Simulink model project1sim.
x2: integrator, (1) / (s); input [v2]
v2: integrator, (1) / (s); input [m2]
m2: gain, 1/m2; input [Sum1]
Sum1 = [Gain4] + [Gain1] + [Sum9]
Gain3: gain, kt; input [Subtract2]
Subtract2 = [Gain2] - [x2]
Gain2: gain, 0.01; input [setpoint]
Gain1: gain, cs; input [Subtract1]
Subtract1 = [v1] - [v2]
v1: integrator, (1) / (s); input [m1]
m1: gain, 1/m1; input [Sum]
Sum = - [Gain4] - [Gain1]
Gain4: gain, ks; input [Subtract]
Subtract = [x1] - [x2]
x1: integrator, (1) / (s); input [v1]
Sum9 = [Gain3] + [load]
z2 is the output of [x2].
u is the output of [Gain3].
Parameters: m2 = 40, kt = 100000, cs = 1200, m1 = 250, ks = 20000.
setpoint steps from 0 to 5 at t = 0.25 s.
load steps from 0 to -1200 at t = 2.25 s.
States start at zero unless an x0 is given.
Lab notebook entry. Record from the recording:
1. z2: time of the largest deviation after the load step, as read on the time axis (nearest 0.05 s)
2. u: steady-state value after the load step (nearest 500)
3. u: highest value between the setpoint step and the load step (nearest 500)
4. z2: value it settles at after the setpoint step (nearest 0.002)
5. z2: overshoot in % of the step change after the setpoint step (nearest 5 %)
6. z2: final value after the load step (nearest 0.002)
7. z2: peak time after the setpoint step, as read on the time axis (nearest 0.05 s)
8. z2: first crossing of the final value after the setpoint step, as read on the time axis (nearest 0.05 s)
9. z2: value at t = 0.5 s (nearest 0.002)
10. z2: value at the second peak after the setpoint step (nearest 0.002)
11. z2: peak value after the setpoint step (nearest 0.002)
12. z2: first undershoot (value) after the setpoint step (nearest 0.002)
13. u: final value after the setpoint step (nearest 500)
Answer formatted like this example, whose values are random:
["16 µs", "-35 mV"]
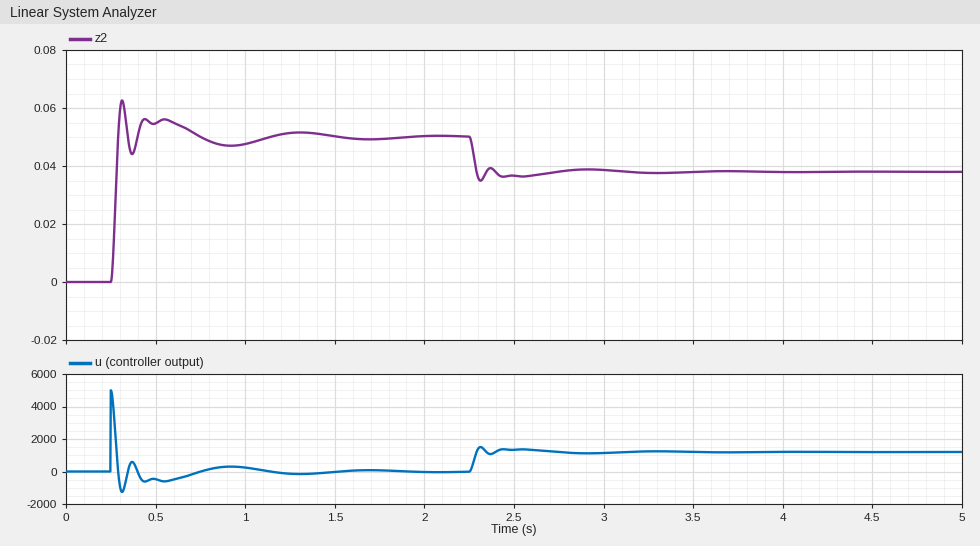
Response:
["2.30 s", "1000", "5000", "0.050", "25 %", "0.038", "0.30 s", "0.30 s", "0.054", "0.056", "0.062", "0.044", "0"]
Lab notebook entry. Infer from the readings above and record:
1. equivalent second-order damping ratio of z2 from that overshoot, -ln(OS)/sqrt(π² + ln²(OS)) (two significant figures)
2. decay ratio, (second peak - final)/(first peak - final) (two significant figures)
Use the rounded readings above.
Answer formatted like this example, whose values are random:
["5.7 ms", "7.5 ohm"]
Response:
["0.40", "0.50"]
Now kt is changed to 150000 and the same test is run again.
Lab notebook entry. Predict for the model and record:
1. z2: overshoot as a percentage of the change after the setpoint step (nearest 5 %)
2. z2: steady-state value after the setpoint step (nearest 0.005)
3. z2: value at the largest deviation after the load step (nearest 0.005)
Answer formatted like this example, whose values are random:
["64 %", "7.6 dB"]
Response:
["35 %", "0.050", "0.040"]
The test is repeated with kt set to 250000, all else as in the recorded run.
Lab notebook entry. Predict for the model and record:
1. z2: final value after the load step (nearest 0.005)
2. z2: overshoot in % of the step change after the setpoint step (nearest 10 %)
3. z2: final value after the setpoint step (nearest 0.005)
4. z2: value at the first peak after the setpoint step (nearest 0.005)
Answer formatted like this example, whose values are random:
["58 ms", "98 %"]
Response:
["0.045", "50 %", "0.050", "0.075"]
